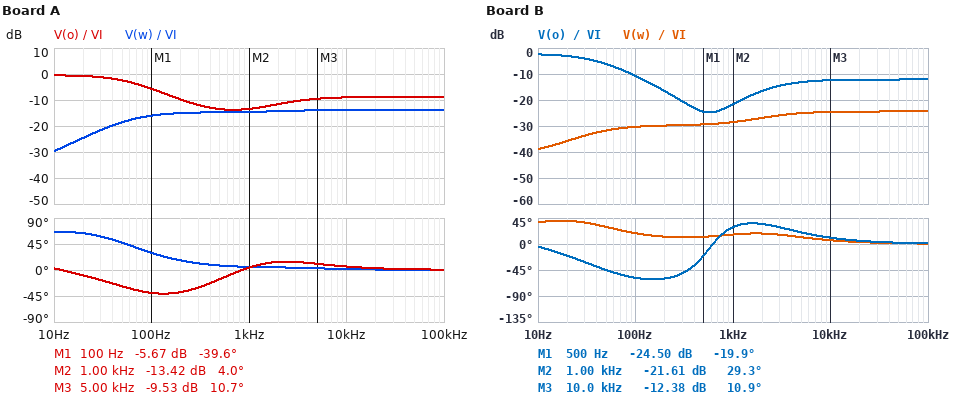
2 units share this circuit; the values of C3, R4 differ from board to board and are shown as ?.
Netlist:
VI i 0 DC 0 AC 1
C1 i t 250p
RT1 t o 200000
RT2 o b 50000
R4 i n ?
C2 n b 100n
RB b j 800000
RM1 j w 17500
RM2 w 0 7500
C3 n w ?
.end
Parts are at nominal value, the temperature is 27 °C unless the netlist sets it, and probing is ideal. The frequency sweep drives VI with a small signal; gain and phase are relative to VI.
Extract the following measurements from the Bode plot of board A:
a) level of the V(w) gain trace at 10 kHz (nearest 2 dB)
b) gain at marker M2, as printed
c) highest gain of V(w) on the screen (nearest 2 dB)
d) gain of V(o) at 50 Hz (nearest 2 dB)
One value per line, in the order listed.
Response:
-14 dB
-13.42 dB
-14 dB
-2 dB
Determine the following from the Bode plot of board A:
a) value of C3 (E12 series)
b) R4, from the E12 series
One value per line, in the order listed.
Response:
68 nF
33 kΩ
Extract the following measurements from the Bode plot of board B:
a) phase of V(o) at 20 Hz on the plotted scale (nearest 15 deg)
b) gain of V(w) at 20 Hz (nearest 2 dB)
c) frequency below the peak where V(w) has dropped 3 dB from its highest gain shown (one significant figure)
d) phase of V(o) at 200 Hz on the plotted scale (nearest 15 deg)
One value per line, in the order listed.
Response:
-15 deg
-36 dB
2 kHz
-60 deg
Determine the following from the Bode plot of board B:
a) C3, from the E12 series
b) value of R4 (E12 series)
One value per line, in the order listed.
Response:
22 nF
220 kΩ
